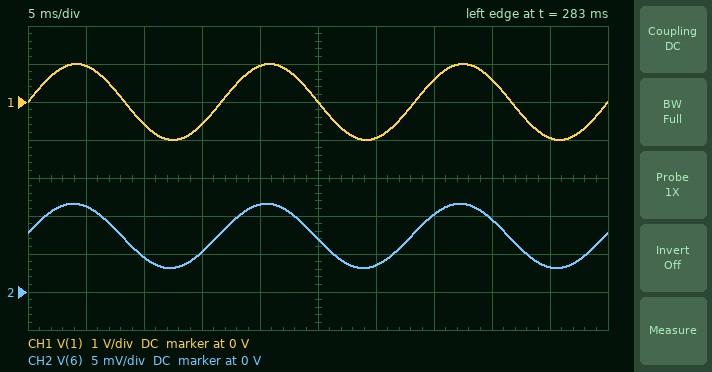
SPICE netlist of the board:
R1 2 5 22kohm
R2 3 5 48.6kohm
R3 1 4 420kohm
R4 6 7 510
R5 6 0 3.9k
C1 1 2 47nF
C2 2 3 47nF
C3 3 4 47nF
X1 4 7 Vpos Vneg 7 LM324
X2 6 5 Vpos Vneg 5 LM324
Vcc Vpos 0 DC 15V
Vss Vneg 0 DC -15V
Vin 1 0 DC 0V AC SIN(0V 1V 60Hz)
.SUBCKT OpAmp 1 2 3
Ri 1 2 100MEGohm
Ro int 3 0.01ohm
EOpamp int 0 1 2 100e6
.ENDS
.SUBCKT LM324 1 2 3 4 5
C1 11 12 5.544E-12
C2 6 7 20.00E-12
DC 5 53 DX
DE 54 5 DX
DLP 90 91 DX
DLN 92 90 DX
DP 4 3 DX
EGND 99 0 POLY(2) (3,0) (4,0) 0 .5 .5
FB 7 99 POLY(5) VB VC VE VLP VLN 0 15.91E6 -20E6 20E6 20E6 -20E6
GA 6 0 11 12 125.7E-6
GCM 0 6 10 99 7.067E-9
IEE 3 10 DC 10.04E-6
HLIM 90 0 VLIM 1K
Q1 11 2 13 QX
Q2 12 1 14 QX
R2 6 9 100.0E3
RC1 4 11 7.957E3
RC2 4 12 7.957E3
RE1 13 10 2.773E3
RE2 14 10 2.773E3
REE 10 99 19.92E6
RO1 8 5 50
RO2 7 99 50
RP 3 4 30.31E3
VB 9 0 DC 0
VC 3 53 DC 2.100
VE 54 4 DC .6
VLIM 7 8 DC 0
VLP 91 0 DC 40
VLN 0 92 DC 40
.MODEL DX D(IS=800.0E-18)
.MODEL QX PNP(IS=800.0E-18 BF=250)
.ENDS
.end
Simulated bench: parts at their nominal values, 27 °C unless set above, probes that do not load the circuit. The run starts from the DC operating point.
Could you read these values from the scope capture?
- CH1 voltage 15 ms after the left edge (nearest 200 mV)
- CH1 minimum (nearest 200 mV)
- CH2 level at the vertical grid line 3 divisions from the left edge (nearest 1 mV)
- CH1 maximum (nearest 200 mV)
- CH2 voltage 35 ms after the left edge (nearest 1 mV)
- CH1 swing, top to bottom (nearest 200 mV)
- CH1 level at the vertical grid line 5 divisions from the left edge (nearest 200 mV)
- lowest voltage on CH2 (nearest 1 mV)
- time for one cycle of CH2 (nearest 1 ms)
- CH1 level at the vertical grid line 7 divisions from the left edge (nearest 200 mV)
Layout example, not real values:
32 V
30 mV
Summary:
-600 mV
-1.0 V
5 mV
1.0 V
10 mV
2.0 V
0 V
3 mV
17 ms
600 mV
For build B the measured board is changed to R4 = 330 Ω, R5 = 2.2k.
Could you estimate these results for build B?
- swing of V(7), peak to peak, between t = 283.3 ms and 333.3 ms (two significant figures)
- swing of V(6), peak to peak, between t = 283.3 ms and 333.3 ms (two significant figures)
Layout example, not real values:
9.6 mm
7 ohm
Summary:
8.5 mV
7.4 mV
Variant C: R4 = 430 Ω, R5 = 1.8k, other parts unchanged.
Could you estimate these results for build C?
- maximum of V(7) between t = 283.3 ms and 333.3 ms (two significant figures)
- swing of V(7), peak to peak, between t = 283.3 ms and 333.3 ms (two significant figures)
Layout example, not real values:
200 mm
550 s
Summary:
11 mV
5.8 mV
